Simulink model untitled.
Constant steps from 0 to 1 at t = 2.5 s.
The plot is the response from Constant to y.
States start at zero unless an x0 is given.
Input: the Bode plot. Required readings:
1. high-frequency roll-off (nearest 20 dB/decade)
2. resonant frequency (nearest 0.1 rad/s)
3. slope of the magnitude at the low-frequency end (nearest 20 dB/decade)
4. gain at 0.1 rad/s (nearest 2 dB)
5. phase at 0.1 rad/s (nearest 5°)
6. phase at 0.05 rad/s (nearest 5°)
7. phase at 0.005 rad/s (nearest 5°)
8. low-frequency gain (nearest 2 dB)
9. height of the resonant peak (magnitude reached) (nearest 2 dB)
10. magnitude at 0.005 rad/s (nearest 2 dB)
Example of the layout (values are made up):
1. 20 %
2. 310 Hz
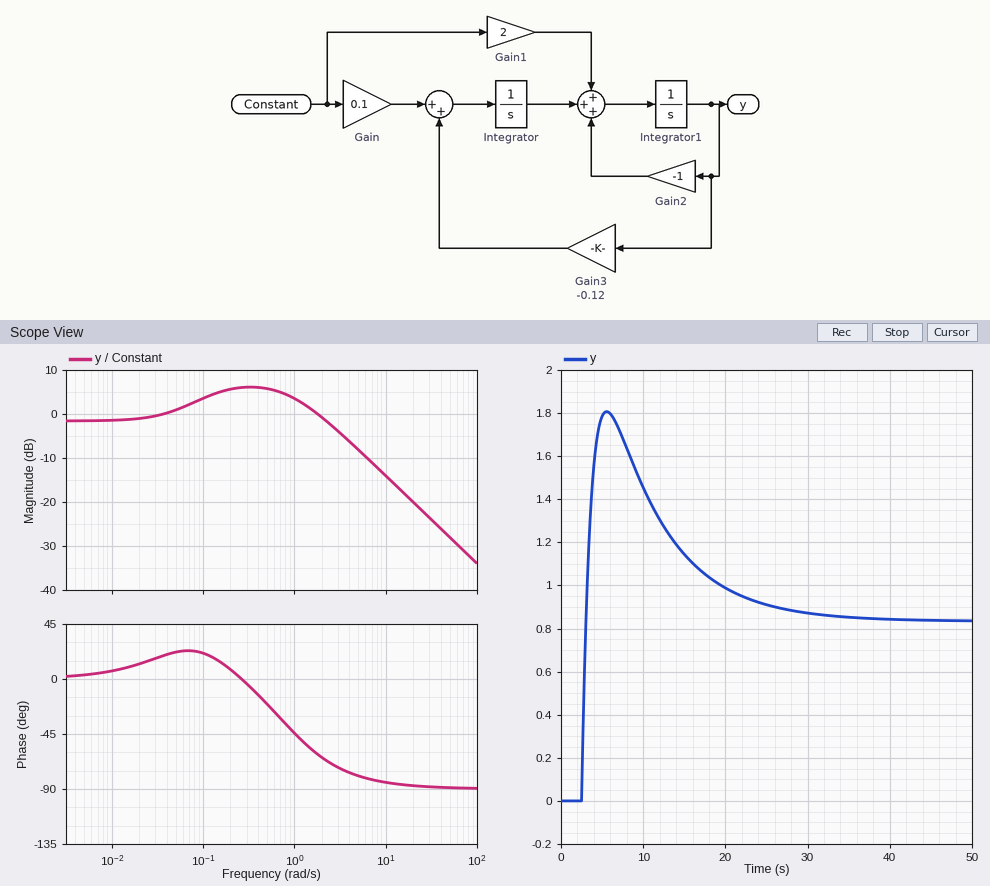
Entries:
1. -20 dB/decade
2. 0.3 rad/s
3. 0 dB/decade
4. 4 dB
5. 20°
6. 20°
7. 5°
8. -2 dB
9. 6 dB
10. -2 dB
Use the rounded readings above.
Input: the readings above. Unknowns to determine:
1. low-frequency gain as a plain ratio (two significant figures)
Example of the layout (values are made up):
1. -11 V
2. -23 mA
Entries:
1. 0.79
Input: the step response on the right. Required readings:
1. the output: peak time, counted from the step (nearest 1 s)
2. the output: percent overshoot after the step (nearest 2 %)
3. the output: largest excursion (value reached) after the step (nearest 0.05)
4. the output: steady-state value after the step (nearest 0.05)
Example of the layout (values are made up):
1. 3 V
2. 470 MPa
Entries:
1. 3 s
2. 116 %
3. 1.80
4. 0.85
